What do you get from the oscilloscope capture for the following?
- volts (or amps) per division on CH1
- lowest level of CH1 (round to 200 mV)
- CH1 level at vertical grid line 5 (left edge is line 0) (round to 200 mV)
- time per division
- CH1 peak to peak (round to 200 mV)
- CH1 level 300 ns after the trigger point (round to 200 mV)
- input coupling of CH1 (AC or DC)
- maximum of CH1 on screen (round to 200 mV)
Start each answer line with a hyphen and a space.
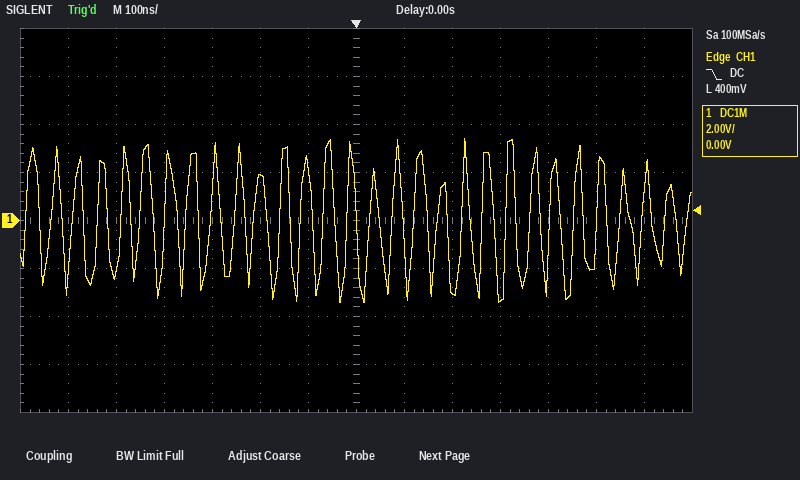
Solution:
- 2 V
- -3.4 V
- 1.8 V
- 100 ns
- 6.8 V
- -3.2 V
- DC
- 3.4 V
